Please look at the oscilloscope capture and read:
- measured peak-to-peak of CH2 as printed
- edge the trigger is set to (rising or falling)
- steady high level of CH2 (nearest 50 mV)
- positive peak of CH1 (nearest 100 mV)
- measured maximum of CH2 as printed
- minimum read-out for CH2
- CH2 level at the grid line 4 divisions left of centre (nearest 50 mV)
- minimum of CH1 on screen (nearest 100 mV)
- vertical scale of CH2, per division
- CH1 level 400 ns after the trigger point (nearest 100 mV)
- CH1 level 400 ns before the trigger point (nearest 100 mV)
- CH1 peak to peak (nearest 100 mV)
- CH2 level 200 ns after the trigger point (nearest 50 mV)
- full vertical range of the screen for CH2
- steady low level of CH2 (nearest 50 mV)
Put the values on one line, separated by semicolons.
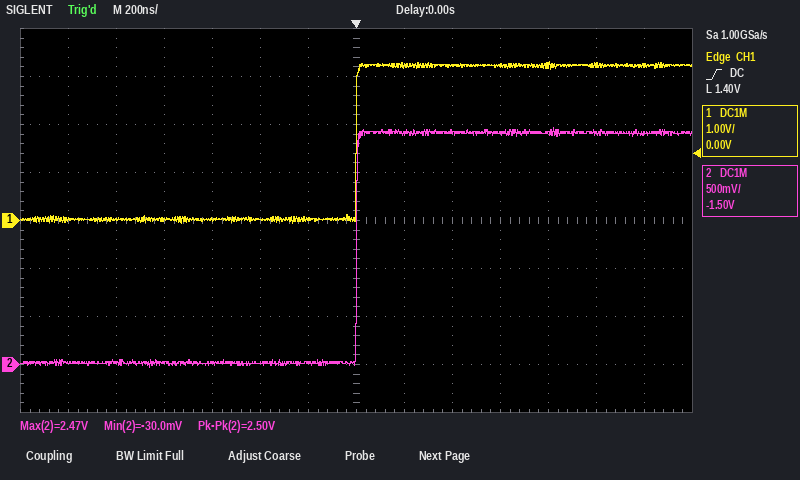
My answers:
2.50 V; rising; 2.40 V; 3.3 V; 2.47 V; -30.0 mV; 0 mV; -100 mV; 500 mV; 3.2 V; 0.0 V; 3.4 V; 2.40 V; 4 V; 0 mV
